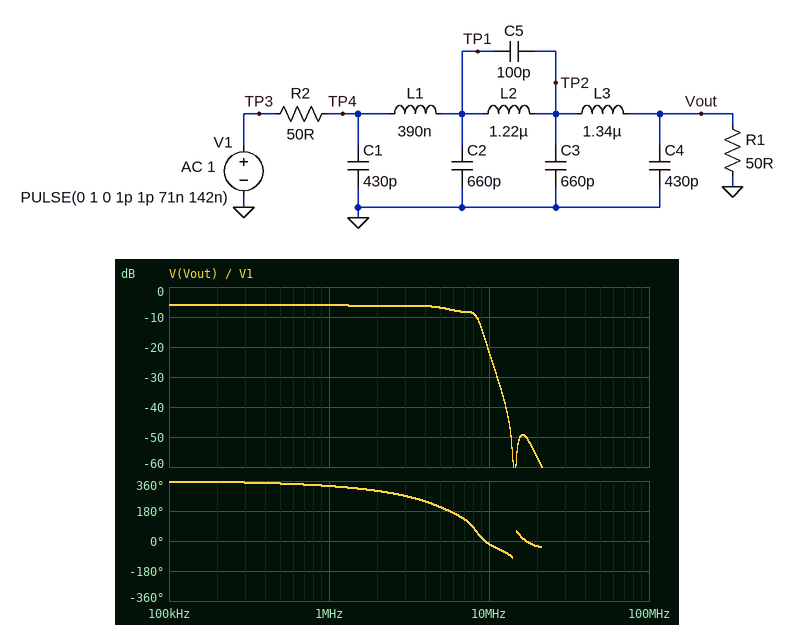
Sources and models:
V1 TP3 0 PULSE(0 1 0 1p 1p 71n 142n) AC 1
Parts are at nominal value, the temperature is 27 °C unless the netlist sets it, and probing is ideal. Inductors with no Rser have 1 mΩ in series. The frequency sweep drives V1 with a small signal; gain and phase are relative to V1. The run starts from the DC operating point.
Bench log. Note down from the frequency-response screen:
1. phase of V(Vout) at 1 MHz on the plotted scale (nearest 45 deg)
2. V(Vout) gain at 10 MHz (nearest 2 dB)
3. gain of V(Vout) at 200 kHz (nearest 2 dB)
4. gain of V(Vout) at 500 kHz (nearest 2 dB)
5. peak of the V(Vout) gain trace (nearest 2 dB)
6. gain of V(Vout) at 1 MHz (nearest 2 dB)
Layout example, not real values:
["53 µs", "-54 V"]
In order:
["315 deg", "-22 dB", "-6 dB", "-6 dB", "-6 dB", "-6 dB"]
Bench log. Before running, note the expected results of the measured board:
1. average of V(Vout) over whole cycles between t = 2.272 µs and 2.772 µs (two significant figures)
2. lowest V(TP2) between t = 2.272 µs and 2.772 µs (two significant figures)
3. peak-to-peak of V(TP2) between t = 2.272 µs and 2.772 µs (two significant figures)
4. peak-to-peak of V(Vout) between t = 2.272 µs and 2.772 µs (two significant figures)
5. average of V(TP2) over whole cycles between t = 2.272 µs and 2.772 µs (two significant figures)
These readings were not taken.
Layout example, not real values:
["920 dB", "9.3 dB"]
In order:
["250 mV", "-45 mV", "590 mV", "490 mV", "250 mV"]
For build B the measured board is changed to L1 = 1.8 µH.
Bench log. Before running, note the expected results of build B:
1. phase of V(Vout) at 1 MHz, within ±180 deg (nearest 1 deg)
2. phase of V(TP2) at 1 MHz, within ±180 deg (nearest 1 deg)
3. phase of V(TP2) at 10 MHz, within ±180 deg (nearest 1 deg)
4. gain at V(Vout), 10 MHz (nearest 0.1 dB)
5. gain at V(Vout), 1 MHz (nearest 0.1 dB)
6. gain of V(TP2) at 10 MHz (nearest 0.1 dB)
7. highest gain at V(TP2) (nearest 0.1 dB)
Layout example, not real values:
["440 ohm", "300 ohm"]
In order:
["-35 deg", "-26 deg", "-22 deg", "-26.4 dB", "-6.0 dB", "-19.9 dB", "-3.6 dB"]
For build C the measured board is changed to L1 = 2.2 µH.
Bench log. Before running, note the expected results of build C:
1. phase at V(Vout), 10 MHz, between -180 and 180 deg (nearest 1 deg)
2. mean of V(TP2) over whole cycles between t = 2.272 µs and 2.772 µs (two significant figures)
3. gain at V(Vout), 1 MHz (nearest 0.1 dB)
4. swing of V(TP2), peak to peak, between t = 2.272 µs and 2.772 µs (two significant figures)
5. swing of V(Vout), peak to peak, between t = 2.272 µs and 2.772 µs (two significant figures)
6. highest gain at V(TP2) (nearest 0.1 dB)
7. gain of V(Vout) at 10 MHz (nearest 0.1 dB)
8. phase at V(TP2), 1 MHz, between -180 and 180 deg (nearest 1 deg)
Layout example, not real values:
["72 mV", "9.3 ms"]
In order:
["-154 deg", "250 mV", "-6.0 dB", "620 mV", "520 mV", "-5.5 dB", "-29.3 dB", "-27 deg"]
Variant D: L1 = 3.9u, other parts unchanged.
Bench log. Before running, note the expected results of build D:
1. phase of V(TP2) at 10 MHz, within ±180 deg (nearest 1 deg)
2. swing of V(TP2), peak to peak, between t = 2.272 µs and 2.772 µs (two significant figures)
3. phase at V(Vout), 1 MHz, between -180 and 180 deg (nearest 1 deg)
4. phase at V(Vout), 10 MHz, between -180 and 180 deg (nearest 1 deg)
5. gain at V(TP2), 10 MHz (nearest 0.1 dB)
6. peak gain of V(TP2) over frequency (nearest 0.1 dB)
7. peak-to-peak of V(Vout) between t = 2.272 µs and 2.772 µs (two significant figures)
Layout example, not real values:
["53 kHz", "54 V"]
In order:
["-34 deg", "320 mV", "-43 deg", "-161 deg", "-29.8 dB", "-6.0 dB", "270 mV"]
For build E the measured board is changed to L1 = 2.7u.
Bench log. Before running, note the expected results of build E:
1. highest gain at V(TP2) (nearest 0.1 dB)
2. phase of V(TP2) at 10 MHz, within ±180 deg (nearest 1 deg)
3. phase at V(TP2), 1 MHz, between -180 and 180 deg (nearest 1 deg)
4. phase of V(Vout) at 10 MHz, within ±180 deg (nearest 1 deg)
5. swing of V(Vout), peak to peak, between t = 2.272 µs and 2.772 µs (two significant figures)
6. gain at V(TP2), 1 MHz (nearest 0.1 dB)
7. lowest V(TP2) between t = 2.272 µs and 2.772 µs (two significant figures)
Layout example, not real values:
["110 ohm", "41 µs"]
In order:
["-6.0 dB", "-31 deg", "-29 deg", "-158 deg", "420 mV", "-6.1 dB", "-2.3 mV"]
